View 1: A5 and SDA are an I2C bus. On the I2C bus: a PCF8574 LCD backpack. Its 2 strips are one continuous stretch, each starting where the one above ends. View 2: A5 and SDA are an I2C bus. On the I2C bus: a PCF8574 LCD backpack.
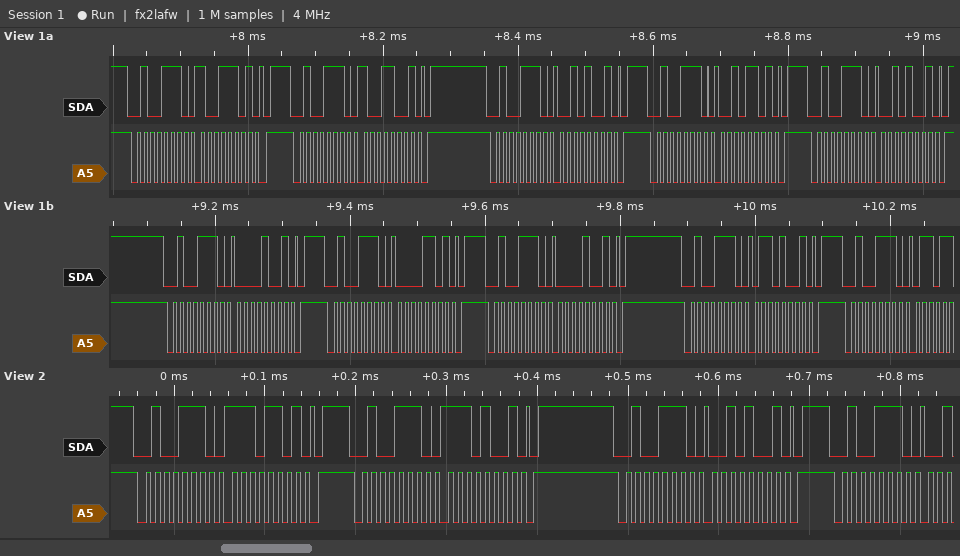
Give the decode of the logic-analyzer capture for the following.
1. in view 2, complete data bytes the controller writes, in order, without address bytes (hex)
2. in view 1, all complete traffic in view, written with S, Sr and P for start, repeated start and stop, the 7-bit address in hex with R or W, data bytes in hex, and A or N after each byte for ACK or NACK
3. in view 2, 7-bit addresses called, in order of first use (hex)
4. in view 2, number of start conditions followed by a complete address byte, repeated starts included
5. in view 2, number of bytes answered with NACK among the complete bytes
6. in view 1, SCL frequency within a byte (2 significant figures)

ED E9 29
S 27W A 9D A P S 27W A 99 A P S 27W A 29 A P S 27W A 2D A P S 27W A 29 A P S 27W A 09 A P S 27W A 0D A P S 27W A 09 A P S 27W A 69 A P S 27W A
0x27
4
0
100 kHz
